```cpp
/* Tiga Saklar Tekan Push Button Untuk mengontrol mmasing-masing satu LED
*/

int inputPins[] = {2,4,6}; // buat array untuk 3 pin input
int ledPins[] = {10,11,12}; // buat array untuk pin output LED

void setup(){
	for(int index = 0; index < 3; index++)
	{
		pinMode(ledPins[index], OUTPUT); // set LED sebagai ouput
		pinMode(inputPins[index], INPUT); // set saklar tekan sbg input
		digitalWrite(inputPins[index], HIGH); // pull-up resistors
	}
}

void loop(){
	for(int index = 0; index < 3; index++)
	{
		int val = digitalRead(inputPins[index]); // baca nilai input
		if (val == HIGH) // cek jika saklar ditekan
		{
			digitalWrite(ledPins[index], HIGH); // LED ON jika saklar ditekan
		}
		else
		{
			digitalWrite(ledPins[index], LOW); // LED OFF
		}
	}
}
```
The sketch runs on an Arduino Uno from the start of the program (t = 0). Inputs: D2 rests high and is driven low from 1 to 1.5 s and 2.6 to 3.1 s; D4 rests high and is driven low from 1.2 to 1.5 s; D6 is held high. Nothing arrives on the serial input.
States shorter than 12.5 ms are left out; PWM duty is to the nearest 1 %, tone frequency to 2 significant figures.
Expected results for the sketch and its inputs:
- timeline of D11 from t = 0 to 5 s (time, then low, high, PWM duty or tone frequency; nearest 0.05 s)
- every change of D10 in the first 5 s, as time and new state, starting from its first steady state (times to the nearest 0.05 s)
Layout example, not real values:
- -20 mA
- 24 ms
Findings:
- 0 s high; 1.2 s low; 1.5 s high
- 0 s high; 1 s low; 1.5 s high; 2.6 s low; 3.1 s high
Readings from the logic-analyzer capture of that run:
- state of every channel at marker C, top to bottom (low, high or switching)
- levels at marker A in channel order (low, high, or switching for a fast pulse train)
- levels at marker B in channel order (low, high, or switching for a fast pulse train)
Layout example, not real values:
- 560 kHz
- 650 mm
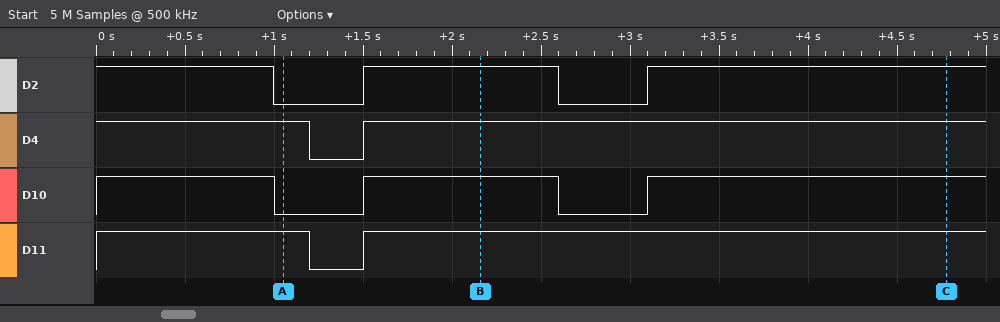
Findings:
- D2 high, D4 high, D10 high, D11 high
- D2 low, D4 high, D10 low, D11 high
- D2 high, D4 high, D10 high, D11 high
